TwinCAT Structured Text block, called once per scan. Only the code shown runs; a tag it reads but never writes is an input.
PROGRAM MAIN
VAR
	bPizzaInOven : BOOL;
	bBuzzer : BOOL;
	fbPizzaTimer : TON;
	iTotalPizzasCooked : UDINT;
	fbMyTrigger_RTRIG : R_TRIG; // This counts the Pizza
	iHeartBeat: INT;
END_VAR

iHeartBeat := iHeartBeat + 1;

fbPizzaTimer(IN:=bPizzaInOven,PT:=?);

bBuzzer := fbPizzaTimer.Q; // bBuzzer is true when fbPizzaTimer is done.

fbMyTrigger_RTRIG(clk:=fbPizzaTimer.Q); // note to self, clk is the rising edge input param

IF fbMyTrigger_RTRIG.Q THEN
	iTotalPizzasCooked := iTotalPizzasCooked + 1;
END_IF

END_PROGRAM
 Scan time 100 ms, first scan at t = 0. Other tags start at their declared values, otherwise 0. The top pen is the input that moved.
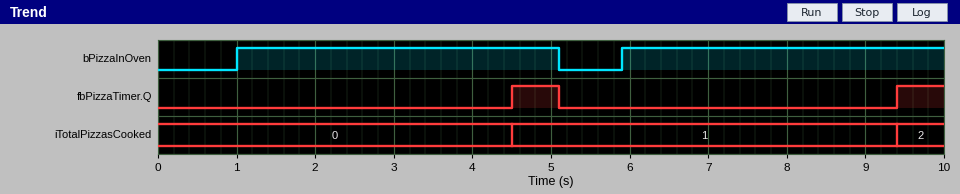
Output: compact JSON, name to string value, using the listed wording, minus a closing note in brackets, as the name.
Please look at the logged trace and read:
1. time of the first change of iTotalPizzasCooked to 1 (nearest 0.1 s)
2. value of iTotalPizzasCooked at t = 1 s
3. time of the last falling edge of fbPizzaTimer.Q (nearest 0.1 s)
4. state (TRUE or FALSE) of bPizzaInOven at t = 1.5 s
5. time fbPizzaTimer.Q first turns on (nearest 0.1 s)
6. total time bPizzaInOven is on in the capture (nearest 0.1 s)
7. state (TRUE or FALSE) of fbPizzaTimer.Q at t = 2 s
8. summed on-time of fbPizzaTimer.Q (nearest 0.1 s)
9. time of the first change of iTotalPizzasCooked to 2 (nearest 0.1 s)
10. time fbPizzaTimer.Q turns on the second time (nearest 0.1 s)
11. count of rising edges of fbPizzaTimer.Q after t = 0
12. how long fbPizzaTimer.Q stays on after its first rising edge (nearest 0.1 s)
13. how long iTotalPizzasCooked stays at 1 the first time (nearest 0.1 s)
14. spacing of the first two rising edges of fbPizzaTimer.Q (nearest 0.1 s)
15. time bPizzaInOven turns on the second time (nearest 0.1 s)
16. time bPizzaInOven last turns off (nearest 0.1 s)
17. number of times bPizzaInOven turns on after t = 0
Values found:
{"time of the first change of iTotalPizzasCooked to 1": "4.5 s", "value of iTotalPizzasCooked at t = 1 s": "0", "time of the last falling edge of fbPizzaTimer.Q": "5.1 s", "state (TRUE or FALSE) of bPizzaInOven at t = 1.5 s": "TRUE", "time fbPizzaTimer.Q first turns on": "4.5 s", "total time bPizzaInOven is on in the capture": "8.2 s", "state (TRUE or FALSE) of fbPizzaTimer.Q at t = 2 s": "FALSE", "summed on-time of fbPizzaTimer.Q": "1.2 s", "time of the first change of iTotalPizzasCooked to 2": "9.4 s", "time fbPizzaTimer.Q turns on the second time": "9.4 s", "count of rising edges of fbPizzaTimer.Q after t = 0": "2", "how long fbPizzaTimer.Q stays on after its first rising edge": "0.6 s", "how long iTotalPizzasCooked stays at 1 the first time": "4.9 s", "spacing of the first two rising edges of fbPizzaTimer.Q": "4.9 s", "time bPizzaInOven turns on the second time": "5.9 s", "time bPizzaInOven last turns off": "5.1 s", "number of times bPizzaInOven turns on after t = 0": "2"}
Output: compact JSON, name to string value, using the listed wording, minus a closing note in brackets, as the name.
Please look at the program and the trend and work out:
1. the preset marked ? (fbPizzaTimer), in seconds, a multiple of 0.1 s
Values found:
{"the preset marked ? (fbPizzaTimer), in seconds, a multiple of 0.1 s": "3.5 s"}
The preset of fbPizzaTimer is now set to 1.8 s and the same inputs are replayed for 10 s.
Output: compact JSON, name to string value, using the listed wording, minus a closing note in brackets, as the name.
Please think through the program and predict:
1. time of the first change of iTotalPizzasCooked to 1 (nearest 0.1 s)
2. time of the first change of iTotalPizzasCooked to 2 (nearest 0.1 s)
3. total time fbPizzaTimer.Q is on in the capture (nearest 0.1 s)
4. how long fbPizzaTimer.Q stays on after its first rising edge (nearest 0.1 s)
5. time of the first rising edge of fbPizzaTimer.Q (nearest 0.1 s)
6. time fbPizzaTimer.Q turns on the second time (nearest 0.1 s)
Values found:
{"time of the first change of iTotalPizzasCooked to 1": "2.8 s", "time of the first change of iTotalPizzasCooked to 2": "7.7 s", "total time fbPizzaTimer.Q is on in the capture": "4.6 s", "how long fbPizzaTimer.Q stays on after its first rising edge": "2.3 s", "time of the first rising edge of fbPizzaTimer.Q": "2.8 s", "time fbPizzaTimer.Q turns on the second time": "7.7 s"}
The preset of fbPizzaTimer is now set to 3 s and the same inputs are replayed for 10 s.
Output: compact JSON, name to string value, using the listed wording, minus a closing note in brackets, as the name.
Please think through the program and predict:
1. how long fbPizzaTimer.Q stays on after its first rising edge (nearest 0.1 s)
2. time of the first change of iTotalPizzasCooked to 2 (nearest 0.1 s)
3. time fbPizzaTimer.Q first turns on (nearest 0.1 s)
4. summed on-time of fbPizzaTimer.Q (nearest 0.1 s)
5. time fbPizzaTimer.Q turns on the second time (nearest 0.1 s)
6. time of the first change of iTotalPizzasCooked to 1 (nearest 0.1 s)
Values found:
{"how long fbPizzaTimer.Q stays on after its first rising edge": "1.1 s", "time of the first change of iTotalPizzasCooked to 2": "8.9 s", "time fbPizzaTimer.Q first turns on": "4.0 s", "summed on-time of fbPizzaTimer.Q": "2.2 s", "time fbPizzaTimer.Q turns on the second time": "8.9 s", "time of the first change of iTotalPizzasCooked to 1": "4.0 s"}
